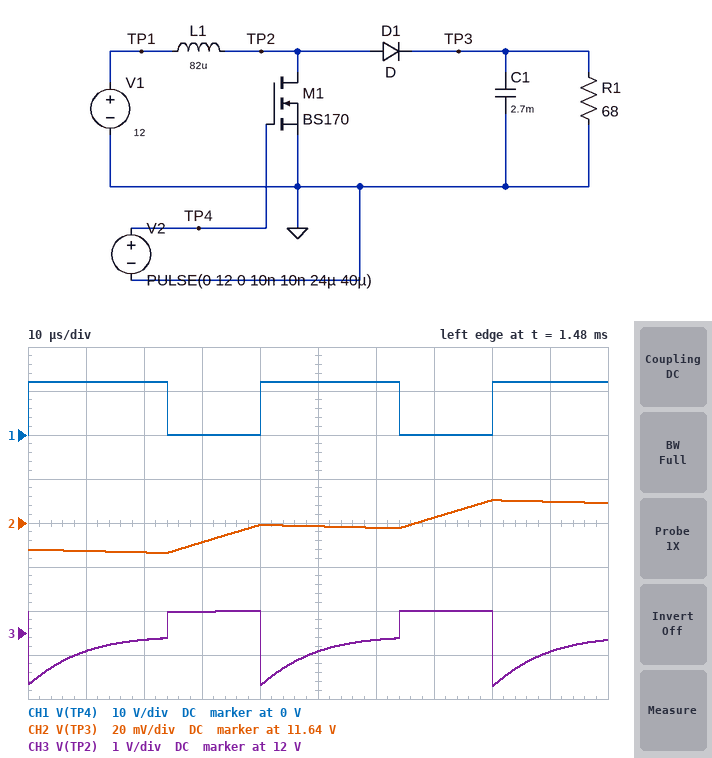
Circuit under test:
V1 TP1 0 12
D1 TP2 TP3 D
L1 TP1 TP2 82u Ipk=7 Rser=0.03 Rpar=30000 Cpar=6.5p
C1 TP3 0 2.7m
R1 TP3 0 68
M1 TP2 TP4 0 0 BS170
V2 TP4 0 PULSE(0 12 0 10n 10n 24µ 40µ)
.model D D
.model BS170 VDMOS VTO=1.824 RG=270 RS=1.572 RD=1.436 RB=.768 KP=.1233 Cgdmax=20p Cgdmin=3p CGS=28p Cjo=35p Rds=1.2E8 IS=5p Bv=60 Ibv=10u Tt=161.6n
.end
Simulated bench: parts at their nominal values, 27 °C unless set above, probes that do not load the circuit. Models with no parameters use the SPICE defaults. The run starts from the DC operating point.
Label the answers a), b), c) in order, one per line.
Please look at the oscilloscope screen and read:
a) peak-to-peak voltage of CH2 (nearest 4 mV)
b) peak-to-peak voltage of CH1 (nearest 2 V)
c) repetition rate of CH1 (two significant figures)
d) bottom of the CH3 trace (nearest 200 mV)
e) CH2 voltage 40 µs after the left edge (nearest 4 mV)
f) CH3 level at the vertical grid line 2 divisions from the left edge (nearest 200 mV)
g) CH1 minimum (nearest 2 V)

a) 24 mV
b) 12 V
c) 25 kHz
d) 10.8 V
e) 11.640 V
f) 11.8 V
g) 0 V
